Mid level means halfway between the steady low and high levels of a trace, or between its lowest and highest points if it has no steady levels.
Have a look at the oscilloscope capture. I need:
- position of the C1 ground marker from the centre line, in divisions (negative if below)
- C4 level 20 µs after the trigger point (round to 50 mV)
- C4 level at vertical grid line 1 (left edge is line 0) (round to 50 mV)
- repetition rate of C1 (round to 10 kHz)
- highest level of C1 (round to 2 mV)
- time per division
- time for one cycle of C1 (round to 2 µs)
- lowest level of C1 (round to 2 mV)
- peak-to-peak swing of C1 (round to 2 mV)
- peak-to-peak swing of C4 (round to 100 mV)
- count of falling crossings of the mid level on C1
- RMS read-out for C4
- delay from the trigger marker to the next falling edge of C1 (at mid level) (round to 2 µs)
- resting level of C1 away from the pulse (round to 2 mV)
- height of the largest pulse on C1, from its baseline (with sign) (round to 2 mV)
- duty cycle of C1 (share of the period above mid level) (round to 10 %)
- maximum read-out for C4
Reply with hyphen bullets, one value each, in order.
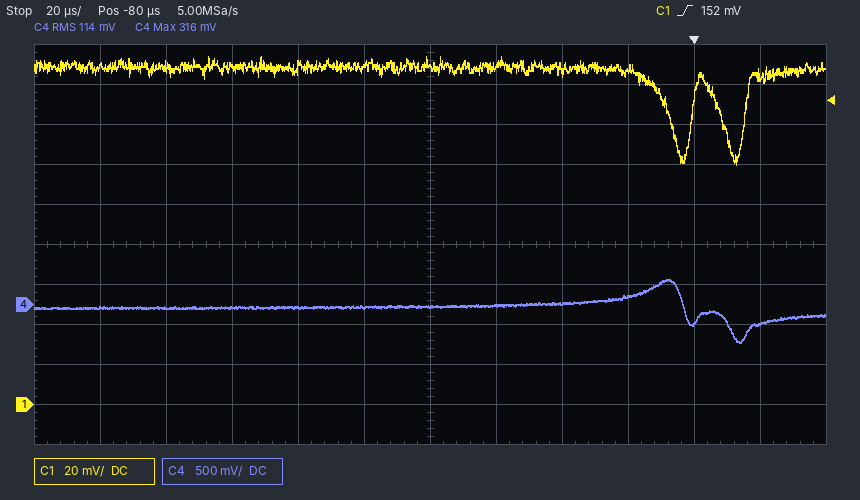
- -4.0 div
- -250 mV
- -50 mV
- 60 kHz
- 174 mV
- 20 µs
- 16 µs
- 120 mV
- 54 mV
- 800 mV
- 2
- 114 mV
- 8 µs
- 168 mV
- -48 mV
- 50 %
- 316 mV
